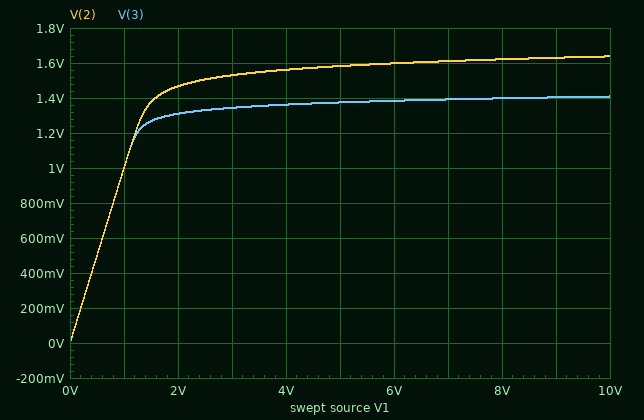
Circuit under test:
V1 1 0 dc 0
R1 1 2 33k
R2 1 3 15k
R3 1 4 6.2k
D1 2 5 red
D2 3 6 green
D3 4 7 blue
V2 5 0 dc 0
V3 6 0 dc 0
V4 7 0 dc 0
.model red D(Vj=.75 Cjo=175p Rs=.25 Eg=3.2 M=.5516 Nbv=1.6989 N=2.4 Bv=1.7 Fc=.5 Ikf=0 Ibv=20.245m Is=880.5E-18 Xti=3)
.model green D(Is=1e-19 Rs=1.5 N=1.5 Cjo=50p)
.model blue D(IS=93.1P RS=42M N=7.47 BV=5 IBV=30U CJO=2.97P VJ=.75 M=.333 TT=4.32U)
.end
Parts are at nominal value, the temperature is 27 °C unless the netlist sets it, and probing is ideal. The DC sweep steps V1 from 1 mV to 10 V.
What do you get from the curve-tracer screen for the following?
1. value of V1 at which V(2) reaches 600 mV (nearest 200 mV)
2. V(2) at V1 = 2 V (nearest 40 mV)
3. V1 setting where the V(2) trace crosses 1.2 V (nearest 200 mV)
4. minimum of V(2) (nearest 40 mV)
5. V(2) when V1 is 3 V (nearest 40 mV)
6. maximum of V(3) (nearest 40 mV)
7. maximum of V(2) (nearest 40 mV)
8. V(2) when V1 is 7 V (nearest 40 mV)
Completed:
600 mV
1.48 V
1.2 V
0 V
1.52 V
1.40 V
1.64 V
1.60 V
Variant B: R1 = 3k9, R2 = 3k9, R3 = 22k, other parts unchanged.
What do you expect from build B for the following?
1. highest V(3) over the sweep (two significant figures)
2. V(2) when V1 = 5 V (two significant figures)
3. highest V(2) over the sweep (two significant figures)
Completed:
1.5 V
1.7 V
1.8 V
